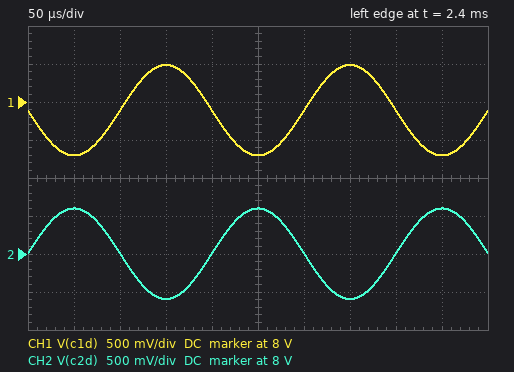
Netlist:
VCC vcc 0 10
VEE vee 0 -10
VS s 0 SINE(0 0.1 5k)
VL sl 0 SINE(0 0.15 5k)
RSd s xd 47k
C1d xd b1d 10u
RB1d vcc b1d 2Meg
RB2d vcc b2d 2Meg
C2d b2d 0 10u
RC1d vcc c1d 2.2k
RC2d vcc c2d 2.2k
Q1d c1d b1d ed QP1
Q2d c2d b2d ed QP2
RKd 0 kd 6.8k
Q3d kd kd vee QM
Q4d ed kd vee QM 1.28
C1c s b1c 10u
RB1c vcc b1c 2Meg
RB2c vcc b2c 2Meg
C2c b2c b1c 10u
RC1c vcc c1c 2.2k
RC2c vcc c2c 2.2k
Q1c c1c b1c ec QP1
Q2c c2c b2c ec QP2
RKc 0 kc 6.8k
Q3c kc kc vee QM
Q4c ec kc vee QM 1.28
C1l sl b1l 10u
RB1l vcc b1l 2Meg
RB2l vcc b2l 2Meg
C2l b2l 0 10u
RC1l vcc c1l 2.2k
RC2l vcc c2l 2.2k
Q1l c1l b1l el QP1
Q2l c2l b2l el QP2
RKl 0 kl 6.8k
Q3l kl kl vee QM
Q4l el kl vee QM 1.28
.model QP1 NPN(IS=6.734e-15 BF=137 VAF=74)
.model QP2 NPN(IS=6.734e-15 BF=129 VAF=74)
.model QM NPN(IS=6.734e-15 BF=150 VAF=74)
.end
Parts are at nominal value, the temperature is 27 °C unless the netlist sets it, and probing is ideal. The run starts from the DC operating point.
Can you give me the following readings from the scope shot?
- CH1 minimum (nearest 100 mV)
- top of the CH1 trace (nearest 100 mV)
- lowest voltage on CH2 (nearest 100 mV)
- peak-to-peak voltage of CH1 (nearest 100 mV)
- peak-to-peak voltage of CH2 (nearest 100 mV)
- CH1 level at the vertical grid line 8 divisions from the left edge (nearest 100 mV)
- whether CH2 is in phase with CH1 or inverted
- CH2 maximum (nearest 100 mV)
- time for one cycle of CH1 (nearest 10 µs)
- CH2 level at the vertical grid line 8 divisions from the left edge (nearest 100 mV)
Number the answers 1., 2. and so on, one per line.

1. 7.3 V
2. 8.5 V
3. 7.4 V
4. 1.2 V
5. 1.2 V
6. 7.9 V
7. inverted
8. 8.6 V
9. 200 µs
10. 8.0 V
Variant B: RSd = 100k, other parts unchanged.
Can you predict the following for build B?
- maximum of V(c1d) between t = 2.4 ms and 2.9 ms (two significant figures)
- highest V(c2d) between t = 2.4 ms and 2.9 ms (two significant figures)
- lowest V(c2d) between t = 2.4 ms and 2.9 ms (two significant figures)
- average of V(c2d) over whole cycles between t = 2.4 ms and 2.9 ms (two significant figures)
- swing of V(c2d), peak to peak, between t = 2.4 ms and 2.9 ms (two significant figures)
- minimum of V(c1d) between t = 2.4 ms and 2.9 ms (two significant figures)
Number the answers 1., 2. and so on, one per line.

1. 8.2 V
2. 8.3 V
3. 7.7 V
4. 8.0 V
5. 610 mV
6. 7.6 V
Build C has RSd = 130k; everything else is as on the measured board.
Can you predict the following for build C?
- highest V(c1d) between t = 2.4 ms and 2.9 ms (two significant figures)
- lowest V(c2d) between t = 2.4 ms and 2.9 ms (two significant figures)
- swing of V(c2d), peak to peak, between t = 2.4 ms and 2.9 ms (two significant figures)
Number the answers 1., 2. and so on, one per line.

1. 8.1 V
2. 7.8 V
3. 480 mV
